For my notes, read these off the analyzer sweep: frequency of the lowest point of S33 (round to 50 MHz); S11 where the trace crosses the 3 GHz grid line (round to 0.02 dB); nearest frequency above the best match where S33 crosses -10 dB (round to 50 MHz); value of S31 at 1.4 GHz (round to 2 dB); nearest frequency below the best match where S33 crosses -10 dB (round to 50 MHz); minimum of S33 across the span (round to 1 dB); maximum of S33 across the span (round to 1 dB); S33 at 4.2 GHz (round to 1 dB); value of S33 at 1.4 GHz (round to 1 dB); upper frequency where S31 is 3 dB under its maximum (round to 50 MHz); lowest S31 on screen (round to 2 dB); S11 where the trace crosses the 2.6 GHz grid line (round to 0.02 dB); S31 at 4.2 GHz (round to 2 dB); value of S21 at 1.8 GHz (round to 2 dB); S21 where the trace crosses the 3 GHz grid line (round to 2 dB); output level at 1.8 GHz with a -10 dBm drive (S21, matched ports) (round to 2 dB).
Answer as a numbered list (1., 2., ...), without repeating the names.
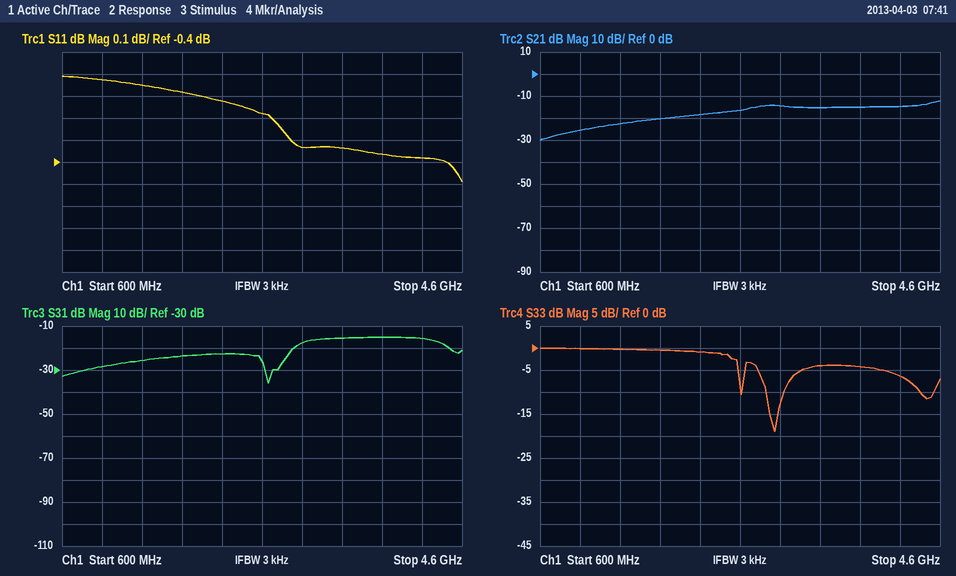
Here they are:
1. 2.95 GHz
2. -0.34 dB
3. 3.05 GHz
4. -26 dB
5. 2.85 GHz
6. -19 dB
7. 0 dB
8. -6 dB
9. 0 dB
10. 4.40 GHz
11. -36 dB
12. -0.18 dB
13. -16 dB
14. -20 dB
15. -14 dB
16. -30 dBm
